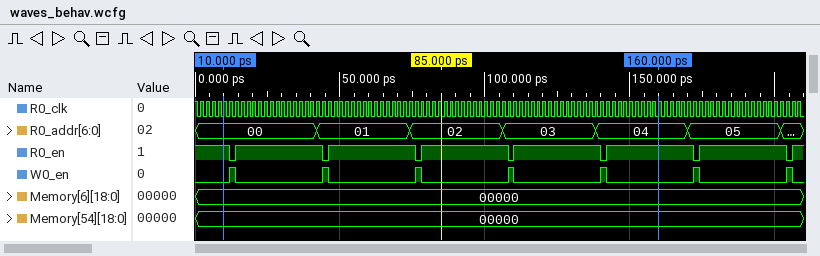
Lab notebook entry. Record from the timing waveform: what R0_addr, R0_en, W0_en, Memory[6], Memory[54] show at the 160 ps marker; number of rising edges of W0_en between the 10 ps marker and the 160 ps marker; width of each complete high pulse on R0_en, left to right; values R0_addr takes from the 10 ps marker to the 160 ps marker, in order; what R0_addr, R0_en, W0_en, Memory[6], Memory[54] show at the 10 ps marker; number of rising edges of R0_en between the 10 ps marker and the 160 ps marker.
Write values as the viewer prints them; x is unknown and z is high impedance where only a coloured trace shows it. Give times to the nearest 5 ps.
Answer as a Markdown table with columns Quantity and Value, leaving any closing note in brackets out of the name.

| Quantity | Value |
|---|---|
| what R0_addr, R0_en, W0_en, Memory[6], Memory[54] show at the 160 ps marker | R0_addr=04, R0_en=1, W0_en=0, Memory[6]=00000, Memory[54]=00000 |
| number of rising edges of W0_en between the 10 ps marker and the 160 ps marker | 5 |
| width of each complete high pulse on R0_en, left to right | 30 ps, 30 ps, 30 ps, 30 ps, 30 ps, 30 ps |
| values R0_addr takes from the 10 ps marker to the 160 ps marker, in order | 00, 01, 02, 03, 04 |
| what R0_addr, R0_en, W0_en, Memory[6], Memory[54] show at the 10 ps marker | R0_addr=00, R0_en=1, W0_en=0, Memory[6]=00000, Memory[54]=00000 |
| number of rising edges of R0_en between the 10 ps marker and the 160 ps marker | 5 |
